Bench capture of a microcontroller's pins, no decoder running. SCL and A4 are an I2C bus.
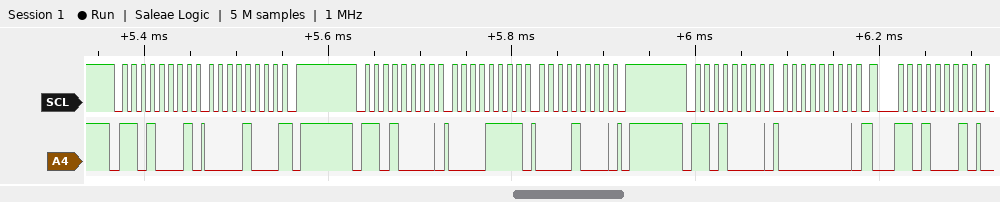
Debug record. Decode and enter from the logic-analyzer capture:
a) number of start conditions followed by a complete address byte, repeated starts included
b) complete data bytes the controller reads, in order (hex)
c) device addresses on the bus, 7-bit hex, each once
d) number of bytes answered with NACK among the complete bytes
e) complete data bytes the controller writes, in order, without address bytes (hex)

4
08
0x68
1
0F 08 00
